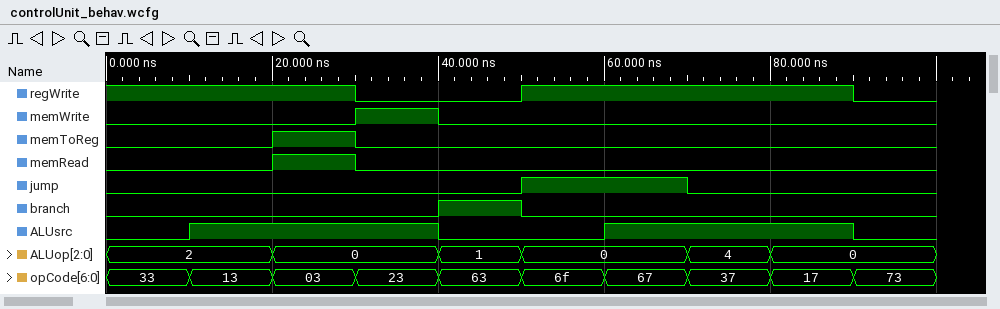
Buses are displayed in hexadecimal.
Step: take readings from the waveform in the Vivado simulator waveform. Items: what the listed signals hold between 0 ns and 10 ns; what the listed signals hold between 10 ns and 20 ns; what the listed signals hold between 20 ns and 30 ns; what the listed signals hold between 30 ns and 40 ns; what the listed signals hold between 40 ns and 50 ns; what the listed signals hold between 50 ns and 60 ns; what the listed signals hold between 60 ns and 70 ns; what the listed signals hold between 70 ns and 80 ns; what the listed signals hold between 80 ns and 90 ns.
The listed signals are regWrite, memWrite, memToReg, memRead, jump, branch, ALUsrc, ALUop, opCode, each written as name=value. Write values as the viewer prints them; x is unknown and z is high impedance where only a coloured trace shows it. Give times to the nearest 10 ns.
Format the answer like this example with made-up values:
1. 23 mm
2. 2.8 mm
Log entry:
1. regWrite=1, memWrite=0, memToReg=0, memRead=0, jump=0, branch=0, ALUsrc=0, ALUop=2, opCode=33
2. regWrite=1, memWrite=0, memToReg=0, memRead=0, jump=0, branch=0, ALUsrc=1, ALUop=2, opCode=13
3. regWrite=1, memWrite=0, memToReg=1, memRead=1, jump=0, branch=0, ALUsrc=1, ALUop=0, opCode=03
4. regWrite=0, memWrite=1, memToReg=0, memRead=0, jump=0, branch=0, ALUsrc=1, ALUop=0, opCode=23
5. regWrite=0, memWrite=0, memToReg=0, memRead=0, jump=0, branch=1, ALUsrc=0, ALUop=1, opCode=63
6. regWrite=1, memWrite=0, memToReg=0, memRead=0, jump=1, branch=0, ALUsrc=0, ALUop=0, opCode=6f
7. regWrite=1, memWrite=0, memToReg=0, memRead=0, jump=1, branch=0, ALUsrc=1, ALUop=0, opCode=67
8. regWrite=1, memWrite=0, memToReg=0, memRead=0, jump=0, branch=0, ALUsrc=1, ALUop=4, opCode=37
9. regWrite=1, memWrite=0, memToReg=0, memRead=0, jump=0, branch=0, ALUsrc=1, ALUop=0, opCode=17
